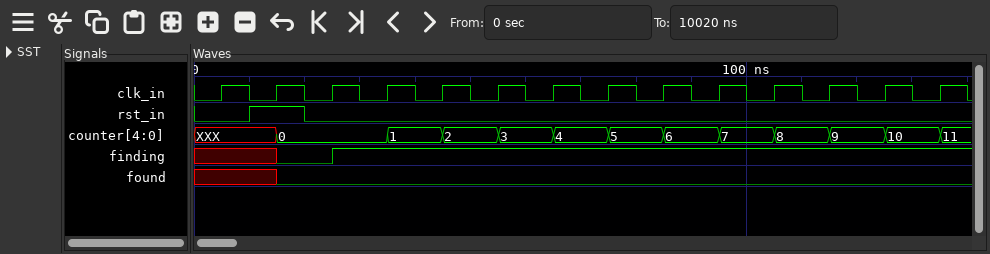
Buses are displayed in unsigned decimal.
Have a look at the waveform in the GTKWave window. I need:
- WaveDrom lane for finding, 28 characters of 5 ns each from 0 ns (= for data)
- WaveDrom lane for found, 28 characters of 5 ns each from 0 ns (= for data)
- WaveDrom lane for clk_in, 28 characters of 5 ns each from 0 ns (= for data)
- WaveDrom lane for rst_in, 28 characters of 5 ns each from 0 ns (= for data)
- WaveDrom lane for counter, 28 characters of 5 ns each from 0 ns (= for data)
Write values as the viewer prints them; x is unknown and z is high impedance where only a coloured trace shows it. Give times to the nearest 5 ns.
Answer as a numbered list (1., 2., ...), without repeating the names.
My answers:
1. {name: 'finding', wave: 'x..0.1......................'}
2. {name: 'found', wave: 'x..0........................'}
3. {name: 'clk_in', wave: '0101010101010101010101010101'}
4. {name: 'rst_in', wave: '0.1.0.......................'}
5. {name: 'counter', wave: 'x..=...=.=.=.=.=.=.=.=.=.=.=', data: '0 1 2 3 4 5 6 7 8 9 10 11'}
